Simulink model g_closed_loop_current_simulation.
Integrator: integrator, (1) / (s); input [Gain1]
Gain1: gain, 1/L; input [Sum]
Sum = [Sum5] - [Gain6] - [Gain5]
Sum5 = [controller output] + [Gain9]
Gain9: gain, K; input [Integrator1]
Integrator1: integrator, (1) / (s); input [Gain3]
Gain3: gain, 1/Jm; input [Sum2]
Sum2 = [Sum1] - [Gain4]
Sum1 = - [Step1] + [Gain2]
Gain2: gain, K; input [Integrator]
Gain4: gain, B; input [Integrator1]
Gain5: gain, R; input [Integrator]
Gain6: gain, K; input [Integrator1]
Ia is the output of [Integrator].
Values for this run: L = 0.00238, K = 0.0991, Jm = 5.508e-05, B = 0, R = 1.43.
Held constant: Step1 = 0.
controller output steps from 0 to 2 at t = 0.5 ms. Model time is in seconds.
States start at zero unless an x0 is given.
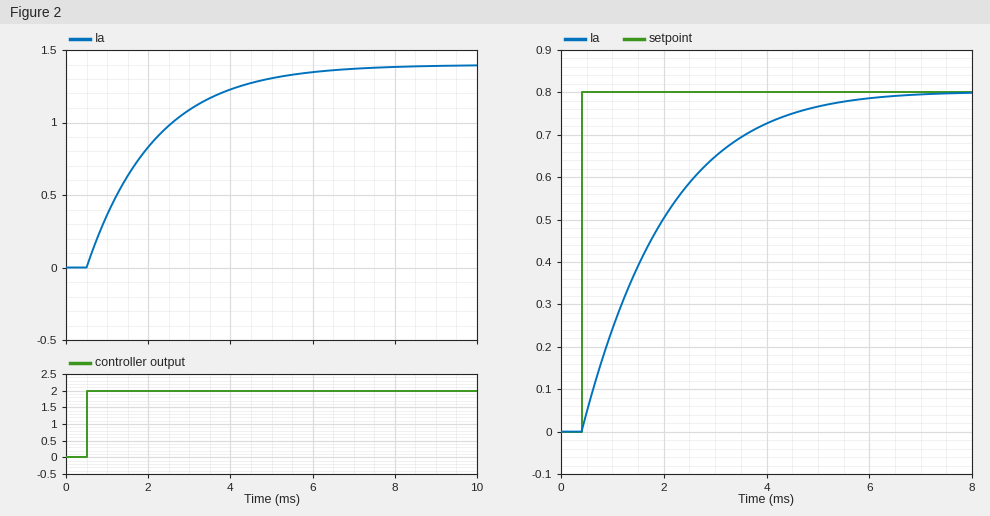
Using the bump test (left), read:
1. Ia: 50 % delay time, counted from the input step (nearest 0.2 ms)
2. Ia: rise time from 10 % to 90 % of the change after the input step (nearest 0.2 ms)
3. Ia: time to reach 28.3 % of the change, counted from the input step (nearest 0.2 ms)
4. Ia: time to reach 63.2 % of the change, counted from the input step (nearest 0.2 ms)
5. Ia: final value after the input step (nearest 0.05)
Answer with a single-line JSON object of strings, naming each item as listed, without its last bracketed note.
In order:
{"Ia: 50 % delay time, counted from the input step": "1.2 ms", "Ia: rise time from 10 % to 90 % of the change after the input step": "3.6 ms", "Ia: time to reach 28.3 % of the change, counted from the input step": "0.6 ms", "Ia: time to reach 63.2 % of the change, counted from the input step": "1.6 ms", "Ia: final value after the input step": "1.40"}
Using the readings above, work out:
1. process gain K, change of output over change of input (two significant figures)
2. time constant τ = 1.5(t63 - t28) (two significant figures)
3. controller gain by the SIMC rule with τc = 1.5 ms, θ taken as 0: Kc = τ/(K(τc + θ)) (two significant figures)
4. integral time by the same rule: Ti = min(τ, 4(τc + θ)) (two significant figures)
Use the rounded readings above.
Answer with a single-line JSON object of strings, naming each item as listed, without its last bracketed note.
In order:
{"process gain K, change of output over change of input": "0.70", "time constant τ = 1.5(t63 - t28)": "1.5 ms", "controller gain by the SIMC rule with τc = 1.5 ms, θ taken as 0: Kc = τ/(K(τc + θ))": "1.4", "integral time by the same rule: Ti = min(τ, 4(τc + θ))": "1.5 ms"}
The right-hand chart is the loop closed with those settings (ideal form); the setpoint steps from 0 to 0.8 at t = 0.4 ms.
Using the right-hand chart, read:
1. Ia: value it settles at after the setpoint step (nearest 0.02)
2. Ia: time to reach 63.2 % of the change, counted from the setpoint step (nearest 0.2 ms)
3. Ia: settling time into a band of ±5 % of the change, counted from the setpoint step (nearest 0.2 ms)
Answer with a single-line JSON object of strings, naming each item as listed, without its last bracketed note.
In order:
{"Ia: value it settles at after the setpoint step": "0.80", "Ia: time to reach 63.2 % of the change, counted from the setpoint step": "1.6 ms", "Ia: settling time into a band of ±5 % of the change, counted from the setpoint step": "4.4 ms"}
